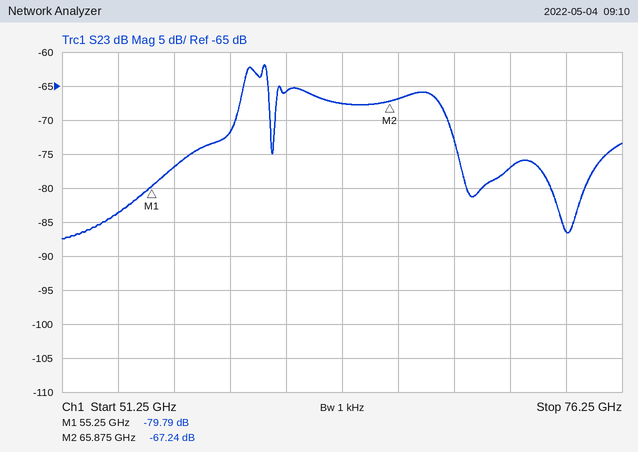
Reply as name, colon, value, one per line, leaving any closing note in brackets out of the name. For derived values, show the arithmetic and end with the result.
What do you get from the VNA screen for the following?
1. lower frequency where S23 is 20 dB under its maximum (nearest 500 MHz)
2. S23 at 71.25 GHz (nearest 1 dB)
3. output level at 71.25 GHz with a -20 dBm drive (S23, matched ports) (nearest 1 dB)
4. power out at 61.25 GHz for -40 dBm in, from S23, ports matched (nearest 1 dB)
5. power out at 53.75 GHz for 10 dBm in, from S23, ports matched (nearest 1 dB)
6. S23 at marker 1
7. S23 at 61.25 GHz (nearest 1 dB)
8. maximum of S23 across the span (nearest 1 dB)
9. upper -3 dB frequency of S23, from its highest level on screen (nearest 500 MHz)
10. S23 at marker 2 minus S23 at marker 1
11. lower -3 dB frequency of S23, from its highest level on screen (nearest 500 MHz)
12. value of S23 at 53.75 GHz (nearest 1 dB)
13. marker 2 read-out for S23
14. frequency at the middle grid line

lower frequency where S23 is 20 dB under its maximum: 54.5 GHz
S23 at 71.25 GHz: -77 dB
output level at 71.25 GHz with a -20 dBm drive (S23, matched ports): -20 dBm + (-77 dB) = -97 dBm
power out at 61.25 GHz for -40 dBm in, from S23, ports matched: -40 dBm + (-66 dB) = -106 dBm
power out at 53.75 GHz for 10 dBm in, from S23, ports matched: 10 dBm + (-84 dB) = -74 dBm
S23 at marker 1: -79.79 dB
S23 at 61.25 GHz: -66 dB
maximum of S23 across the span: -62 dB
upper -3 dB frequency of S23, from its highest level on screen: 60.5 GHz
S23 at marker 2 minus S23 at marker 1: -67.24 − (-79.79) = 12.55 dB
lower -3 dB frequency of S23, from its highest level on screen: 59.5 GHz
value of S23 at 53.75 GHz: -84 dB
marker 2 read-out for S23: -67.24 dB
frequency at the middle grid line: 63.75 GHz
